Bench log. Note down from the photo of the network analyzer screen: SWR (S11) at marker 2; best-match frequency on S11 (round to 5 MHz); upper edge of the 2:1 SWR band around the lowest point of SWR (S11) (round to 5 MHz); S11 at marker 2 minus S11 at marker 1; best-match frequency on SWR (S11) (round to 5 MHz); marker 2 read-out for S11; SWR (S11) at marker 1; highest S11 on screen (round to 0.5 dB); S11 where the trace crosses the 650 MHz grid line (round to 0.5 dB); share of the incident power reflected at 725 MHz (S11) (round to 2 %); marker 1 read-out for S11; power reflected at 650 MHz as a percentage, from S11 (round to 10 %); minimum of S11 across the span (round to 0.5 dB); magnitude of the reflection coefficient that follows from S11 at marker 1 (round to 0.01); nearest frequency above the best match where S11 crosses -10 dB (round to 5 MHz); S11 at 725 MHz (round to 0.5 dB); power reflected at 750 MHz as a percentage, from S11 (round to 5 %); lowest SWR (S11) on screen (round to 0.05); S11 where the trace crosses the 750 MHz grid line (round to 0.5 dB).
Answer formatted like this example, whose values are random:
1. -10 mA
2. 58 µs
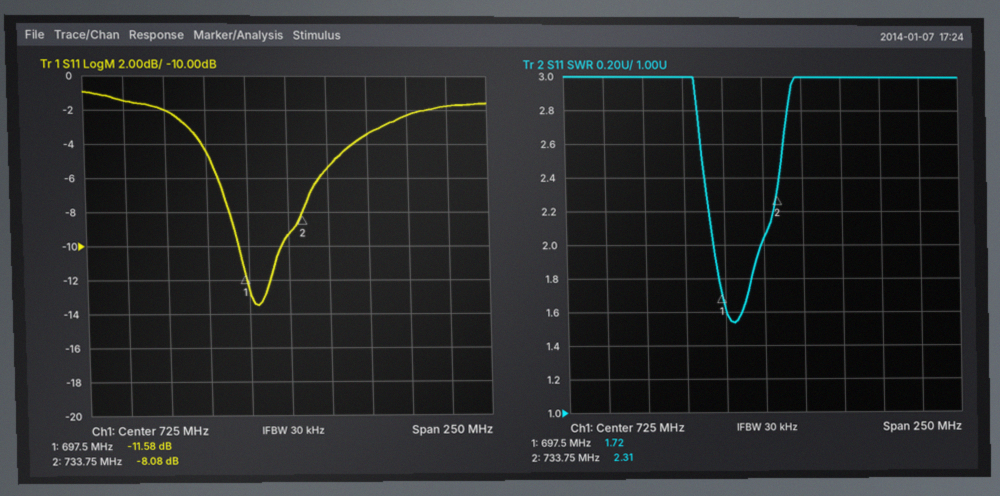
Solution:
1. 2.31
2. 705 MHz
3. 725 MHz
4. 3.50 dB
5. 705 MHz
6. -8.08 dB
7. 1.72
8. -1.0 dB
9. -2.0 dB
10. 12 %
11. -11.58 dB
12. 60 %
13. -13.5 dB
14. 0.26
15. 720 MHz
16. -9.5 dB
17. 30 %
18. 1.55
19. -5.5 dB
